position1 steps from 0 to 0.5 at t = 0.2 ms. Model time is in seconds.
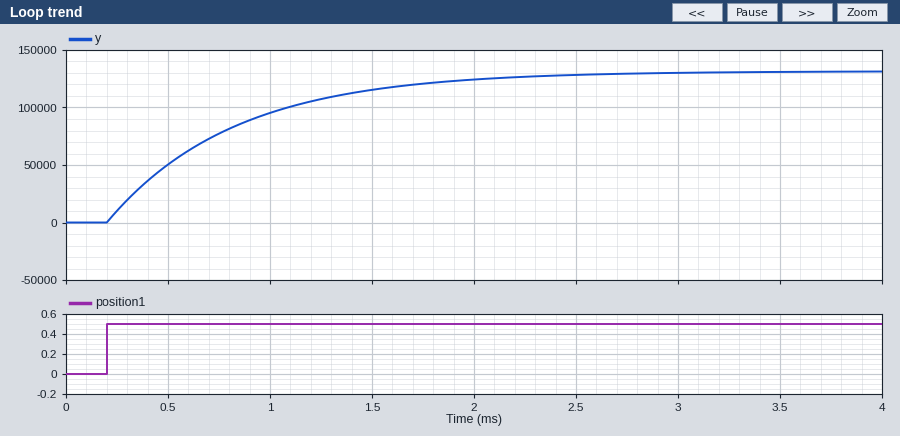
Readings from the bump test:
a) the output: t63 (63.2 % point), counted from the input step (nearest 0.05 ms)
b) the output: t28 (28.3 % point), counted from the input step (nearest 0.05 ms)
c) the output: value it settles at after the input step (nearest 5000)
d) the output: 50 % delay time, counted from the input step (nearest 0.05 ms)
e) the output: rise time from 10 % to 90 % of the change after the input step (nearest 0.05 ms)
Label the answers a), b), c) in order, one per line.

a) 0.60 ms
b) 0.20 ms
c) 130000
d) 0.45 ms
e) 1.35 ms
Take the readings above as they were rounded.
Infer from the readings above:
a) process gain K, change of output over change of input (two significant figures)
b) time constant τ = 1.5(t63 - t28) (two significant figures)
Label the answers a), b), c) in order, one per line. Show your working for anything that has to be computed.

a) (130000 - 0) / 0.5 = 260000
b) 1.5 × (0.6 - 0.2) = 0.60 ms
